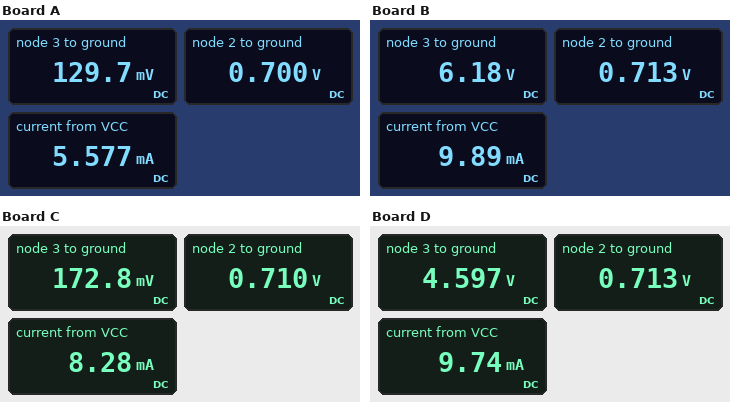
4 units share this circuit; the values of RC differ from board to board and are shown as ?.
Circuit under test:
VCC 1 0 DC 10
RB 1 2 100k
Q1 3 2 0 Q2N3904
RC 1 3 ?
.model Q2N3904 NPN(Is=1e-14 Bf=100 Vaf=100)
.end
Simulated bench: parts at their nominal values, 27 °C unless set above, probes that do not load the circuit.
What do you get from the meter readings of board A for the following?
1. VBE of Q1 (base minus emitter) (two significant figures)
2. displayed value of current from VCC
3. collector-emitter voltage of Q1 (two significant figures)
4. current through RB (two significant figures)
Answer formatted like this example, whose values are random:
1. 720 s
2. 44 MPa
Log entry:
1. 700 mV
2. 5.577 mA
3. 130 mV
4. 93 µA
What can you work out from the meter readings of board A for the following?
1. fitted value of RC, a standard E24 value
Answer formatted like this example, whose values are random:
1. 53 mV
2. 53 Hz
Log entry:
1. 1.8 kΩ
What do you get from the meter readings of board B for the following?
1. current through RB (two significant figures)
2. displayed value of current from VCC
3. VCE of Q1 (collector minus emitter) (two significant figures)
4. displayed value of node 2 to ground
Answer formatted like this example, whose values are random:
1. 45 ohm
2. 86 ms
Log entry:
1. 93 µA
2. 9.89 mA
3. 6.2 V
4. 0.713 V
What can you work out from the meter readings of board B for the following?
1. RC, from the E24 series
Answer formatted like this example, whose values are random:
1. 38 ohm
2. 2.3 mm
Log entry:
1. 390 Ω
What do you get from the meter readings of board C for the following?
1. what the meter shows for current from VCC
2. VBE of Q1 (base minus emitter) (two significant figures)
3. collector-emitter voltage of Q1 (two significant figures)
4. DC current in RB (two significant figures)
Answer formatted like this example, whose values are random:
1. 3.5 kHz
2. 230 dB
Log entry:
1. 8.28 mA
2. 710 mV
3. 170 mV
4. 93 µA
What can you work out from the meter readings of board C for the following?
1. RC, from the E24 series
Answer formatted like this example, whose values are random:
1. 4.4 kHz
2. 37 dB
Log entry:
1. 1.2 kΩ
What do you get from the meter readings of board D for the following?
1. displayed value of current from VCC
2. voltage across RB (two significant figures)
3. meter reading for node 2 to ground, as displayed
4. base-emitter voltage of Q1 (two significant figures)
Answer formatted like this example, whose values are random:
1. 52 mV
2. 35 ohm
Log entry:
1. 9.74 mA
2. 9.3 V
3. 0.713 V
4. 710 mV
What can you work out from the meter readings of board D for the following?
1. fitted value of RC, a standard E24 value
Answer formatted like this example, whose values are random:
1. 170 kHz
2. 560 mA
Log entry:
1. 560 Ω
